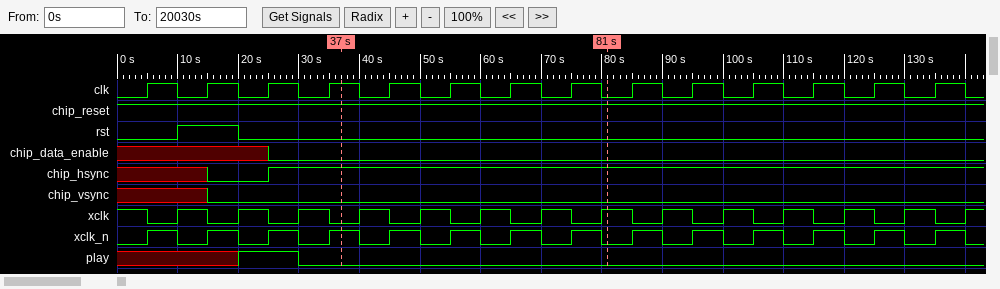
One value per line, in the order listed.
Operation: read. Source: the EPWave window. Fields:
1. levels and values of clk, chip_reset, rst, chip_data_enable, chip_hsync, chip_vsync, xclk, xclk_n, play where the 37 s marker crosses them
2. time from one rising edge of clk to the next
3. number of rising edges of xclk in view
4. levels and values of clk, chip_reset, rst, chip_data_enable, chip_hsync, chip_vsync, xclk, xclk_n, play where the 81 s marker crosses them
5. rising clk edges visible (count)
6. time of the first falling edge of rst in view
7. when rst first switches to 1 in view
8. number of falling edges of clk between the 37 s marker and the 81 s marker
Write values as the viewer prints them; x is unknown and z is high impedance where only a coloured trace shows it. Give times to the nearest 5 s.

clk=1, chip_reset=1, rst=0, chip_data_enable=0, chip_hsync=1, chip_vsync=0, xclk=0, xclk_n=1, play=0
10 s
14
clk=0, chip_reset=1, rst=0, chip_data_enable=0, chip_hsync=1, chip_vsync=0, xclk=1, xclk_n=0, play=0
14
20 s
10 s
5
